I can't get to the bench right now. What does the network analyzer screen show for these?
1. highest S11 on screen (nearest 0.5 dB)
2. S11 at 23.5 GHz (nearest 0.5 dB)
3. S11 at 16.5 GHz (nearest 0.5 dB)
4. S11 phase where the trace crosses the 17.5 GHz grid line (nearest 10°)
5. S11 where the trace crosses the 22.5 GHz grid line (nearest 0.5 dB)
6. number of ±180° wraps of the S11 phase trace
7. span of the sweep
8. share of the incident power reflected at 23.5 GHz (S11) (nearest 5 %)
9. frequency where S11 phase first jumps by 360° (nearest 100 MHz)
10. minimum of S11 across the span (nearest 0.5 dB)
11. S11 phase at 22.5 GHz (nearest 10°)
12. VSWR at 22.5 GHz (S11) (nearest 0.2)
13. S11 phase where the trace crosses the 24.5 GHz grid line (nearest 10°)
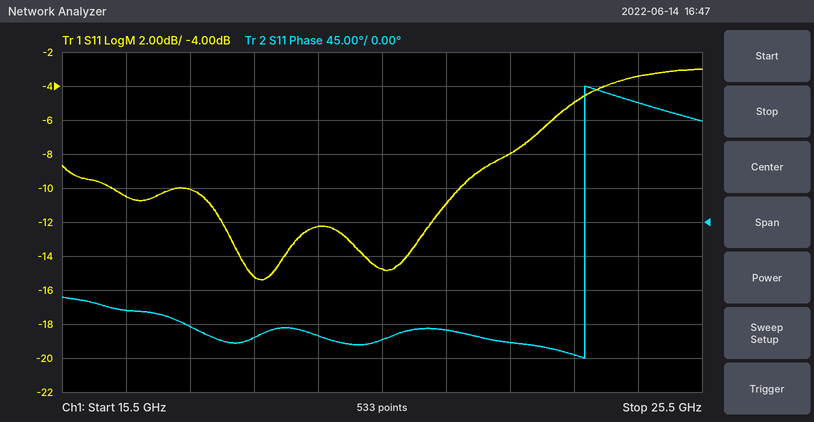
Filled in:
-3.0 dB
-5.0 dB
-10.5 dB
-140°
-8.0 dB
1
10 GHz
30 %
23.7 GHz
-15.5 dB
-160°
2.4
160°
